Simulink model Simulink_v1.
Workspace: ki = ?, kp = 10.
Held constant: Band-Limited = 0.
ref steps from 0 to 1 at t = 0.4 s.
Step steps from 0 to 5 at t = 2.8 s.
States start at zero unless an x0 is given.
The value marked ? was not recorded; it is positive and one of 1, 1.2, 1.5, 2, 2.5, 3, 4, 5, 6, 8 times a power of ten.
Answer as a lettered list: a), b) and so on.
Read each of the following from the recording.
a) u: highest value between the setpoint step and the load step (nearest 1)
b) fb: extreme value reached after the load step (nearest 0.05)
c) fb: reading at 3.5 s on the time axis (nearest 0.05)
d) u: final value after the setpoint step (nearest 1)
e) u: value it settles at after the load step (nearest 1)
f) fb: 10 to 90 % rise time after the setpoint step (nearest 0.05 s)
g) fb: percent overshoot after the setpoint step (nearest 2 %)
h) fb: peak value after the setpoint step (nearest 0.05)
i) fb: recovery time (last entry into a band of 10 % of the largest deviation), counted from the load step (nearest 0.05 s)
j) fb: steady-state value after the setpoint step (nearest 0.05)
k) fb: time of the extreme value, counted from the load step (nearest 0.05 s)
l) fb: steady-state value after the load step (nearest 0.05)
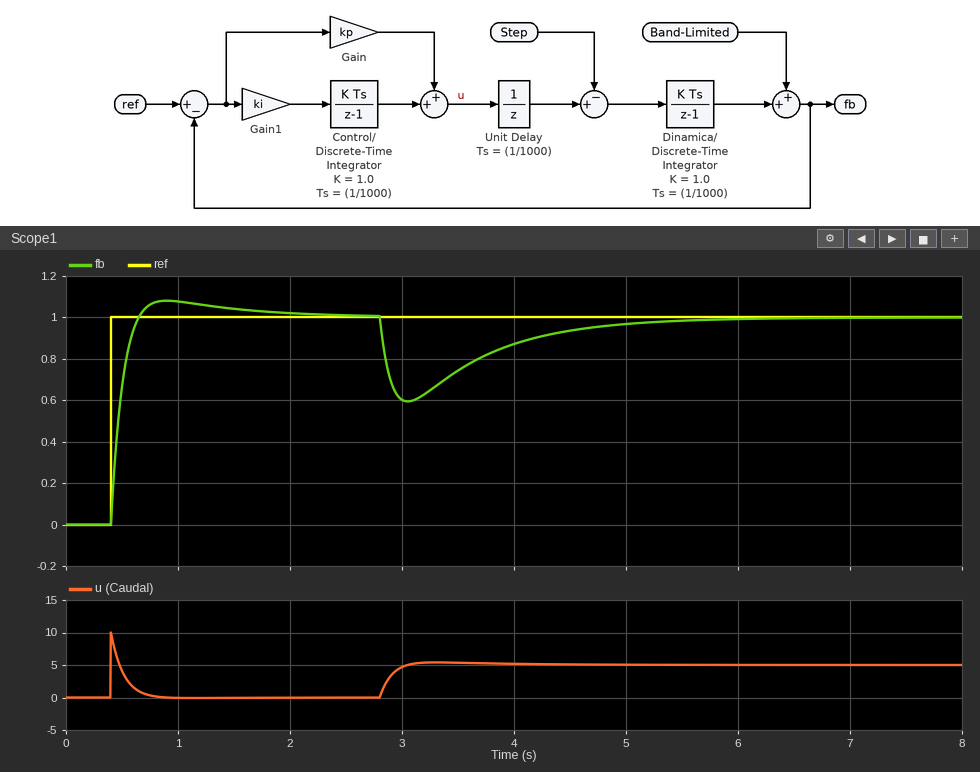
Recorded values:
a) 10
b) 0.60
c) 0.75
d) 0
e) 5
f) 0.15 s
g) 8 %
h) 1.10
i) 2.00 s
j) 1.00
k) 0.25 s
l) 1.00
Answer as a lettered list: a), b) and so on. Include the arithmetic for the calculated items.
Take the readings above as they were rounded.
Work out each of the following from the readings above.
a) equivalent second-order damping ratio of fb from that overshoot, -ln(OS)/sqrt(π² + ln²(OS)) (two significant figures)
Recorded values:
a) ln(0.08) = -2.526; 2.526 / sqrt(9.870 + 6.379) = 0.63
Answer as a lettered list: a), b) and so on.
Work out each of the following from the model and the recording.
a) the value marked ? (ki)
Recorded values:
a) 12
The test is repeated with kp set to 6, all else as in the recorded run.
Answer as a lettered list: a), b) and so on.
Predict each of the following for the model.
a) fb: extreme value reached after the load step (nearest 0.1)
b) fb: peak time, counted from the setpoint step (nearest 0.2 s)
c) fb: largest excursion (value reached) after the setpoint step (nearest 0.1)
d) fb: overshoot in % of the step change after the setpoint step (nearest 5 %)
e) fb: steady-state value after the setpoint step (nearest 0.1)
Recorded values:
a) 0.4
b) 0.6 s
c) 1.2
d) 15 %
e) 1.0
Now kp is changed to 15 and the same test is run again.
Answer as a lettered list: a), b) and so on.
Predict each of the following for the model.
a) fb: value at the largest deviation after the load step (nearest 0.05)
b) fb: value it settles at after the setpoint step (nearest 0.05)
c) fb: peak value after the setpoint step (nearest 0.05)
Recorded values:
a) 0.70
b) 1.00
c) 1.05
